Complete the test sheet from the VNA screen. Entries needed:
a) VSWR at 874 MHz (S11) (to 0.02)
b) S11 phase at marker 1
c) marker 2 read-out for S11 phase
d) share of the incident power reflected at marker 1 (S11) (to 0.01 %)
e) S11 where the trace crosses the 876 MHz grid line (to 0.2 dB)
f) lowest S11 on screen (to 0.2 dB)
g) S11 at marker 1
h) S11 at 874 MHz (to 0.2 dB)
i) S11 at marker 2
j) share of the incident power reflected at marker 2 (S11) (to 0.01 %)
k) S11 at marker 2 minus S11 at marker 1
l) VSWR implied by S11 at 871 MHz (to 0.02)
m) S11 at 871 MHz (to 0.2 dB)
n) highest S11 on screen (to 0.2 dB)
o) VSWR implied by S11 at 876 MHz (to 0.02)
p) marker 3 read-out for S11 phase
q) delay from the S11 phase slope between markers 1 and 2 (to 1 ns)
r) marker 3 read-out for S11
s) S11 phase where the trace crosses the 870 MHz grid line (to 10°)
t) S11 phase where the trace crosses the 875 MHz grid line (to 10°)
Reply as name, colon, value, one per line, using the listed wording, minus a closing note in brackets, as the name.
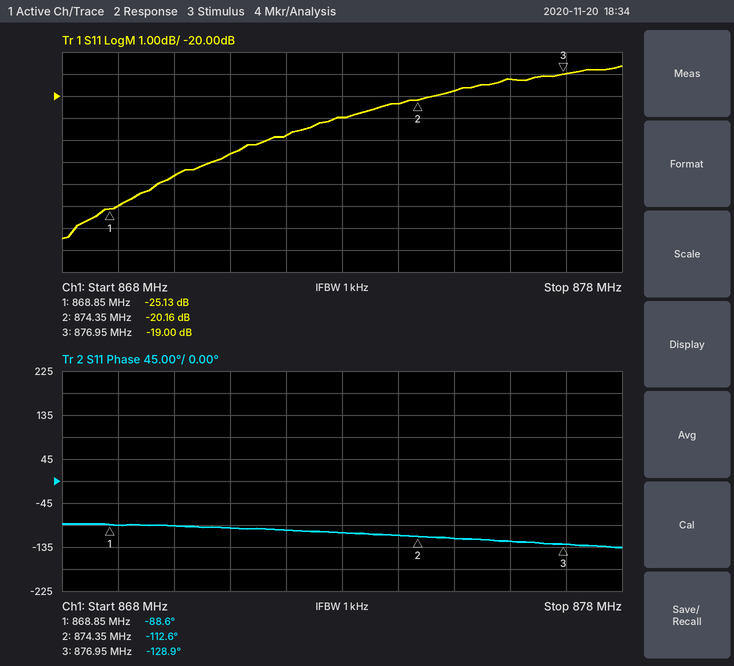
VSWR at 874 MHz (S11): 1.22
S11 phase at marker 1: -88.6°
marker 2 read-out for S11 phase: -112.6°
share of the incident power reflected at marker 1 (S11): 0.31 %
S11 where the trace crosses the 876 MHz grid line: -19.2 dB
lowest S11 on screen: -26.4 dB
S11 at marker 1: -25.13 dB
S11 at 874 MHz: -20.4 dB
S11 at marker 2: -20.16 dB
share of the incident power reflected at marker 2 (S11): 0.96 %
S11 at marker 2 minus S11 at marker 1: 4.97 dB
VSWR implied by S11 at 871 MHz: 1.16
S11 at 871 MHz: -22.6 dB
highest S11 on screen: -18.6 dB
VSWR implied by S11 at 876 MHz: 1.24
marker 3 read-out for S11 phase: -128.9°
delay from the S11 phase slope between markers 1 and 2: 12 ns
marker 3 read-out for S11: -19.00 dB
S11 phase where the trace crosses the 870 MHz grid line: -90°
S11 phase where the trace crosses the 875 MHz grid line: -120°
